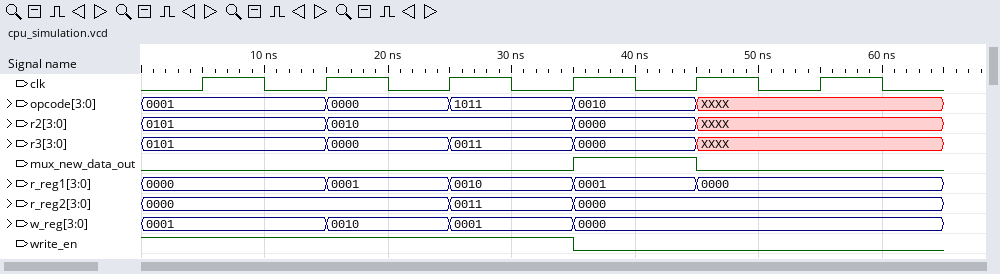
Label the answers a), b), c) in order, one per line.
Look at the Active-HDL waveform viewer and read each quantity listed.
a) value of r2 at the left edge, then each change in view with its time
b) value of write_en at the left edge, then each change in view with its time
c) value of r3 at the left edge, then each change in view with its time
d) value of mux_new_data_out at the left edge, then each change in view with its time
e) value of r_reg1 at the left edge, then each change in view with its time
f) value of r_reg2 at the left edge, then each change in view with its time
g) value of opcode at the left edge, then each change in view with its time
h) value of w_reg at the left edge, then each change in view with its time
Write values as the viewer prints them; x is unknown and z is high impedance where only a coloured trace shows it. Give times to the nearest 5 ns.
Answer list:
a) 0101, 0010 at 15 ns, 0000 at 35 ns, XXXX at 45 ns
b) 1, 0 at 35 ns
c) 0101, 0000 at 15 ns, 0011 at 25 ns, 0000 at 35 ns, XXXX at 45 ns
d) 0, 1 at 35 ns, 0 at 45 ns
e) 0000, 0001 at 15 ns, 0010 at 25 ns, 0001 at 35 ns, 0000 at 45 ns
f) 0000, 0011 at 25 ns, 0000 at 35 ns
g) 0001, 0000 at 15 ns, 1011 at 25 ns, 0010 at 35 ns, XXXX at 45 ns
h) 0001, 0010 at 15 ns, 0001 at 25 ns, 0000 at 35 ns
